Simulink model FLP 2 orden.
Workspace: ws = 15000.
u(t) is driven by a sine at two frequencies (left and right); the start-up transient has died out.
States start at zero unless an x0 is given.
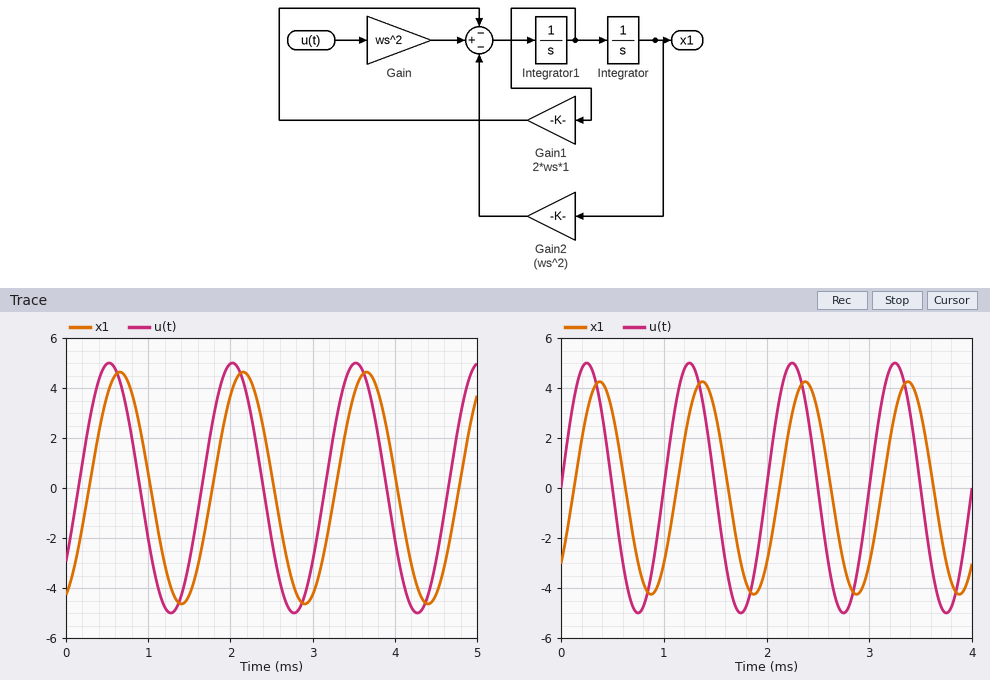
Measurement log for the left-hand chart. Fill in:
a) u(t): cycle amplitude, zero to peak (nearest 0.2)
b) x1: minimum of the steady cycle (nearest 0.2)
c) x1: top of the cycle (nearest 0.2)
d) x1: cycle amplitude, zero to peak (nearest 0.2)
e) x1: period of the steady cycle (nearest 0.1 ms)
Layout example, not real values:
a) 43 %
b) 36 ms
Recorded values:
a) 5.0
b) -4.6
c) 4.6
d) 4.6
e) 1.5 ms
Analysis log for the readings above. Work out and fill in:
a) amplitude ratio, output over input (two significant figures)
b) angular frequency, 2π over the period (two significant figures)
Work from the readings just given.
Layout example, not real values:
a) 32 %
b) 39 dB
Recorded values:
a) 0.92
b) 4.2 rad/ms
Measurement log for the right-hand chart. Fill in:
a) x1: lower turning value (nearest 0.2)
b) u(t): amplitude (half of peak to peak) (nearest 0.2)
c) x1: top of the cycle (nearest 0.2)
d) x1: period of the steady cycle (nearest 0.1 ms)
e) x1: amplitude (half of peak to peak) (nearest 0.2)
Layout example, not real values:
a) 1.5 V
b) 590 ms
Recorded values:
a) -4.2
b) 5.0
c) 4.2
d) 1.0 ms
e) 4.2
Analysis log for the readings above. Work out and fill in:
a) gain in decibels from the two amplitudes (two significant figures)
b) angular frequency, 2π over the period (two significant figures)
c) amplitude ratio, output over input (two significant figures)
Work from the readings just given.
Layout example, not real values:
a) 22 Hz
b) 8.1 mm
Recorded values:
a) -1.5 dB
b) 6.3 rad/ms
c) 0.84
